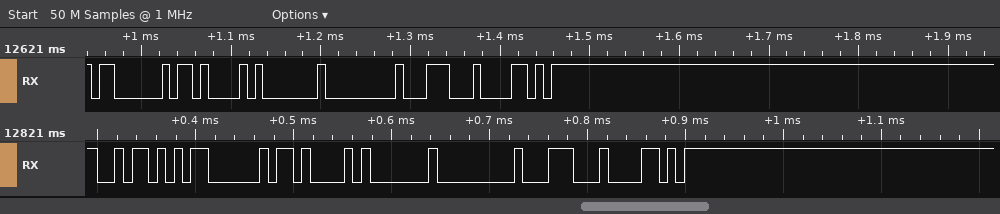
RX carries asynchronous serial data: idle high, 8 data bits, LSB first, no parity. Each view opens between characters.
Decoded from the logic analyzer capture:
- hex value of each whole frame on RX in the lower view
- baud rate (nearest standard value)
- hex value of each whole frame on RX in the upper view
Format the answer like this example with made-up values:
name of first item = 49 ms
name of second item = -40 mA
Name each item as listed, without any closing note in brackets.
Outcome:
hex value of each whole frame on RX in the lower view = 5A, 03, 0B, 01, 00, 1C, 58
baud rate = 115200 baud
hex value of each whole frame on RX in the upper view = 03, 0B, 01, 00, 1C, 58
